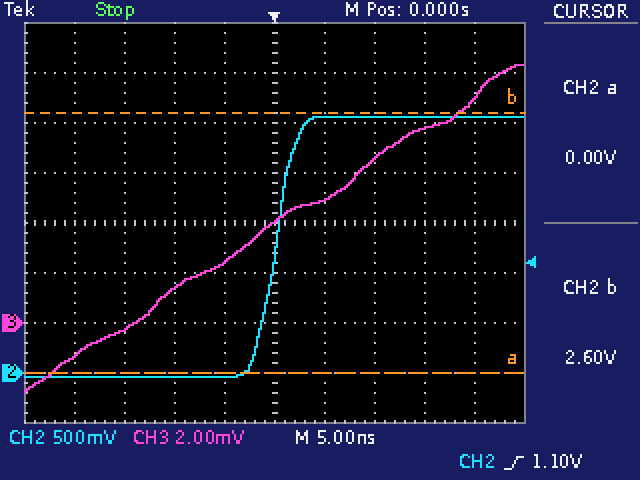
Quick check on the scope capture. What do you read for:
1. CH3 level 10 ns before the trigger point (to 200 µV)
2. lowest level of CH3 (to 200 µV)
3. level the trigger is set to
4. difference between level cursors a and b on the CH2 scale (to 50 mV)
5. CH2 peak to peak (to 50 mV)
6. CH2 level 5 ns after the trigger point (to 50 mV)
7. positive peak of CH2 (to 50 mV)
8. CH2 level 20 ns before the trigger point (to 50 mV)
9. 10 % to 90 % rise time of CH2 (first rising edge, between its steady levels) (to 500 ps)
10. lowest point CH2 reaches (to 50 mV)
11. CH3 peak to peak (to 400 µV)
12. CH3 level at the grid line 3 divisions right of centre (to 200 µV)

1.4 mV
-2.8 mV
1.10 V
2.60 V
2.60 V
2.55 V
2.55 V
-50 mV
4.0 ns
-50 mV
13.2 mV
7.8 mV
